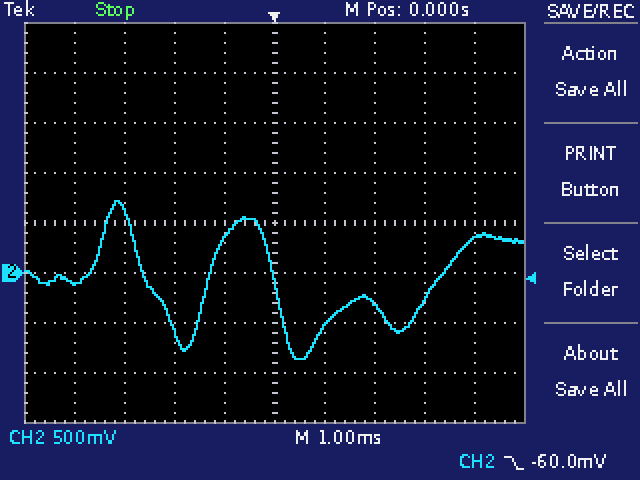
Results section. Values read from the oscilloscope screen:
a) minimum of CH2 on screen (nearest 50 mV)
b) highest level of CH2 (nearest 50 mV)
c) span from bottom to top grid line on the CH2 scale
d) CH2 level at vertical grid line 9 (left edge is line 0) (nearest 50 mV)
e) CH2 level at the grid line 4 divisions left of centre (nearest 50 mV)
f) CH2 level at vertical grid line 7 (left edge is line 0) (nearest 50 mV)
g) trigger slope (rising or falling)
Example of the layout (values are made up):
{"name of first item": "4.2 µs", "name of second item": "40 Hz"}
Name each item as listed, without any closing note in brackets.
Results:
{"minimum of CH2 on screen": "-850 mV", "highest level of CH2": "700 mV", "span from bottom to top grid line on the CH2 scale": "4 V", "CH2 level at vertical grid line 9 (left edge is line 0)": "350 mV", "CH2 level at the grid line 4 divisions left of centre": "-100 mV", "CH2 level at vertical grid line 7 (left edge is line 0)": "-300 mV", "trigger slope": "falling"}
